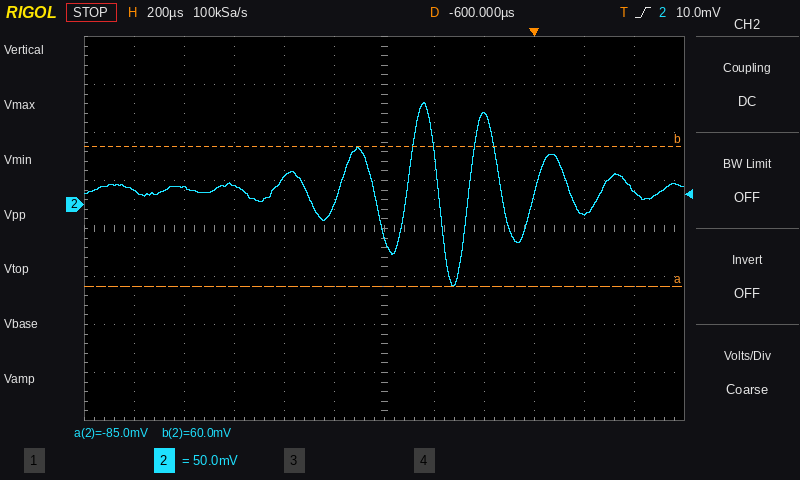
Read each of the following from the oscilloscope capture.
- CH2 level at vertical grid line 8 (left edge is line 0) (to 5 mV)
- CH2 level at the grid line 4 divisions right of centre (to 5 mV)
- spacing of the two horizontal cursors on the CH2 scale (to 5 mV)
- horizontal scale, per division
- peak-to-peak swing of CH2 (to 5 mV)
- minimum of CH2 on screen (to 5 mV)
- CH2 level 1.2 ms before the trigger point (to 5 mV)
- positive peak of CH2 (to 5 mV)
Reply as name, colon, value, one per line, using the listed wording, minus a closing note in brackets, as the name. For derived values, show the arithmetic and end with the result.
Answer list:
CH2 level at vertical grid line 8 (left edge is line 0): 95 mV
CH2 level at the grid line 4 divisions right of centre: -10 mV
spacing of the two horizontal cursors on the CH2 scale: 145 mV
horizontal scale, per division: 200 µs
peak-to-peak swing of CH2: 105 mV − (-85 mV) = 190 mV
minimum of CH2 on screen: -85 mV
CH2 level 1.2 ms before the trigger point: 20 mV
positive peak of CH2: 105 mV
